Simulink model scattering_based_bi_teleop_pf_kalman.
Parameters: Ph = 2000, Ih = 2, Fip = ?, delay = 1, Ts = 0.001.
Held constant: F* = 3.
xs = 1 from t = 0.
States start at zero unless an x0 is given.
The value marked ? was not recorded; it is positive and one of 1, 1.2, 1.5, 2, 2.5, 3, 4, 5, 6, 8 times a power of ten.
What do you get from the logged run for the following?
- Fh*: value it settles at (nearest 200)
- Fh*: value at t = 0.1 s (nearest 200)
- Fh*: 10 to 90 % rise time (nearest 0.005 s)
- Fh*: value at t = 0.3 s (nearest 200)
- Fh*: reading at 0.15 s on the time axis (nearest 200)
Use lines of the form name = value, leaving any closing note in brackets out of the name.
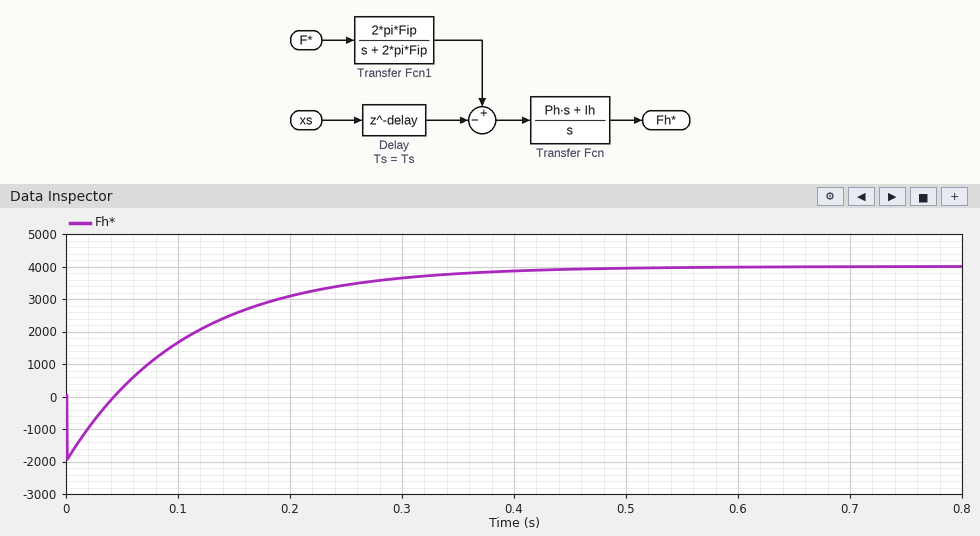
Fh*: value it settles at = 4000
Fh*: value at t = 0.1 s = 1600
Fh*: 10 to 90 % rise time = 0.235 s
Fh*: value at t = 0.3 s = 3600
Fh*: reading at 0.15 s on the time axis = 2600
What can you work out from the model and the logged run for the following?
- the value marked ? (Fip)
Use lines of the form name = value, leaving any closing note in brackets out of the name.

the value marked ? = 1.5
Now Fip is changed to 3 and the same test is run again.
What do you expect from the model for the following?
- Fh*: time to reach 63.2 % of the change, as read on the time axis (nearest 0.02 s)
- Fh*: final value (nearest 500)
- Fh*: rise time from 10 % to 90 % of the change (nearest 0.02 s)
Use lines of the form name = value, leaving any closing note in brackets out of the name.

Fh*: time to reach 63.2 % of the change, as read on the time axis = 0.08 s
Fh*: final value = 4000
Fh*: rise time from 10 % to 90 % of the change = 0.12 s
